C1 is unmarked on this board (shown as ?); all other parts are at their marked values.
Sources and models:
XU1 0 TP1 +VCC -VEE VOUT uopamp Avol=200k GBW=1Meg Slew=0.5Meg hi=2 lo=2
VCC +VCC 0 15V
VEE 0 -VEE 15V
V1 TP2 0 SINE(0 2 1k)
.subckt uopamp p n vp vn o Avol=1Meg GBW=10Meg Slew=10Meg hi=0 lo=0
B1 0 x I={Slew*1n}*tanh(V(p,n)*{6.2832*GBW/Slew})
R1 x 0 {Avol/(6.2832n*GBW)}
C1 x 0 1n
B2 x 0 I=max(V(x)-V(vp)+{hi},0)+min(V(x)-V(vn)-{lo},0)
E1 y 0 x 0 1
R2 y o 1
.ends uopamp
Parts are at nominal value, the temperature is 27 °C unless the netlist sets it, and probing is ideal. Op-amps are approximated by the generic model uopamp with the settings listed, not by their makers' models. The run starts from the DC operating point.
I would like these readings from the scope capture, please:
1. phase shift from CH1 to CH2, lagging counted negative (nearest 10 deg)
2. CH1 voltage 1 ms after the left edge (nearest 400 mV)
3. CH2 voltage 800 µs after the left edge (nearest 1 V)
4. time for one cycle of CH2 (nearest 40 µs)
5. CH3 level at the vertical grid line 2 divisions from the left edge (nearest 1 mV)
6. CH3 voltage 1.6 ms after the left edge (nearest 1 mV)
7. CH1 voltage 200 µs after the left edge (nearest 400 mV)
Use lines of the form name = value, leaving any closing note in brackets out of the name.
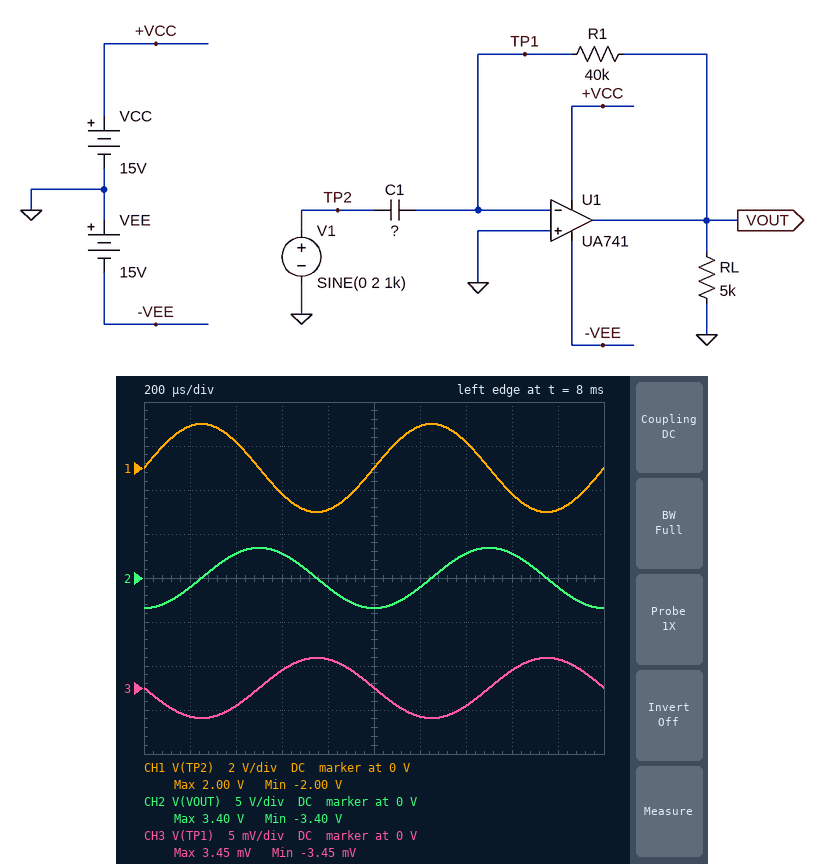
phase shift from CH1 to CH2, lagging counted negative = -90 deg
CH1 voltage 1 ms after the left edge = 0 V
CH2 voltage 800 µs after the left edge = -1 V
time for one cycle of CH2 = 1.00 ms
CH3 level at the vertical grid line 2 divisions from the left edge = -2 mV
CH3 voltage 1.6 ms after the left edge = 2 mV
CH1 voltage 200 µs after the left edge = 2.0 V
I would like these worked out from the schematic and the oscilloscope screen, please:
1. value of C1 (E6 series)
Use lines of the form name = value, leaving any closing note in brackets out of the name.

value of C1 = 6.8 nF
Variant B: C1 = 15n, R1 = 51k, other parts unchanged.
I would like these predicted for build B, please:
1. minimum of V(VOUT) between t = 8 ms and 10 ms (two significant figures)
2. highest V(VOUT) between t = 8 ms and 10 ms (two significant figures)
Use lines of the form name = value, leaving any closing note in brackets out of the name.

minimum of V(VOUT) between t = 8 ms and 10 ms = -9.7 V
highest V(VOUT) between t = 8 ms and 10 ms = 9.7 V
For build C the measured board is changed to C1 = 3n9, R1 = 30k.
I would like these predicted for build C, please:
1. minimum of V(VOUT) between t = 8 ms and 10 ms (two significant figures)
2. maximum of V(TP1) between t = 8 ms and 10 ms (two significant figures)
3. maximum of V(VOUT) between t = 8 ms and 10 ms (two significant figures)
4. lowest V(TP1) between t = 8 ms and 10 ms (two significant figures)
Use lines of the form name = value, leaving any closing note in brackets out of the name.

minimum of V(VOUT) between t = 8 ms and 10 ms = -1.5 V
maximum of V(TP1) between t = 8 ms and 10 ms = 1.5 mV
maximum of V(VOUT) between t = 8 ms and 10 ms = 1.5 V
lowest V(TP1) between t = 8 ms and 10 ms = -1.5 mV
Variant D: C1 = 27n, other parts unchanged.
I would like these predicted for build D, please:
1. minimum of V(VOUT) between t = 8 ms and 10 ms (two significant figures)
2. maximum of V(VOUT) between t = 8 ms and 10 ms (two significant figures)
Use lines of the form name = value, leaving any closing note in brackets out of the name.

minimum of V(VOUT) between t = 8 ms and 10 ms = -13 V
maximum of V(VOUT) between t = 8 ms and 10 ms = 13 V
